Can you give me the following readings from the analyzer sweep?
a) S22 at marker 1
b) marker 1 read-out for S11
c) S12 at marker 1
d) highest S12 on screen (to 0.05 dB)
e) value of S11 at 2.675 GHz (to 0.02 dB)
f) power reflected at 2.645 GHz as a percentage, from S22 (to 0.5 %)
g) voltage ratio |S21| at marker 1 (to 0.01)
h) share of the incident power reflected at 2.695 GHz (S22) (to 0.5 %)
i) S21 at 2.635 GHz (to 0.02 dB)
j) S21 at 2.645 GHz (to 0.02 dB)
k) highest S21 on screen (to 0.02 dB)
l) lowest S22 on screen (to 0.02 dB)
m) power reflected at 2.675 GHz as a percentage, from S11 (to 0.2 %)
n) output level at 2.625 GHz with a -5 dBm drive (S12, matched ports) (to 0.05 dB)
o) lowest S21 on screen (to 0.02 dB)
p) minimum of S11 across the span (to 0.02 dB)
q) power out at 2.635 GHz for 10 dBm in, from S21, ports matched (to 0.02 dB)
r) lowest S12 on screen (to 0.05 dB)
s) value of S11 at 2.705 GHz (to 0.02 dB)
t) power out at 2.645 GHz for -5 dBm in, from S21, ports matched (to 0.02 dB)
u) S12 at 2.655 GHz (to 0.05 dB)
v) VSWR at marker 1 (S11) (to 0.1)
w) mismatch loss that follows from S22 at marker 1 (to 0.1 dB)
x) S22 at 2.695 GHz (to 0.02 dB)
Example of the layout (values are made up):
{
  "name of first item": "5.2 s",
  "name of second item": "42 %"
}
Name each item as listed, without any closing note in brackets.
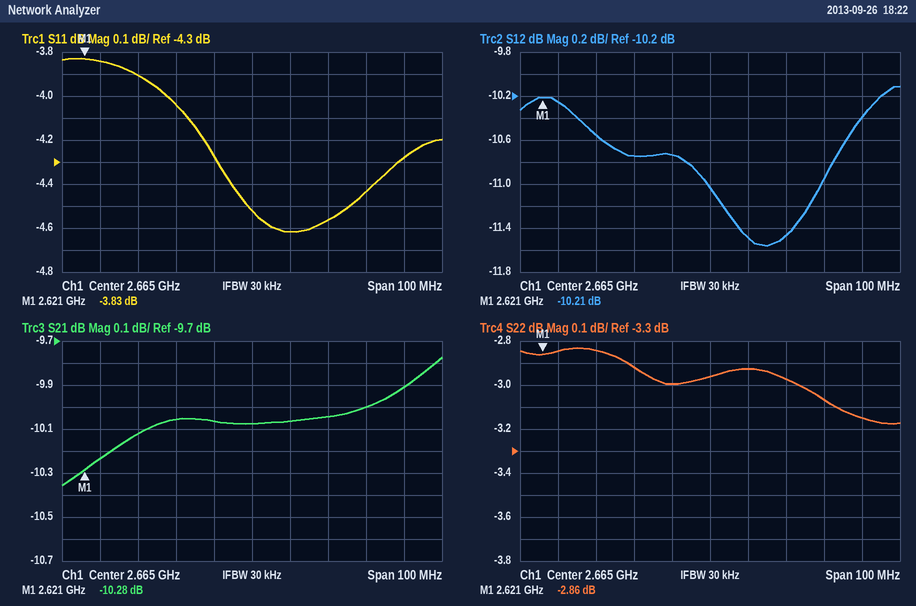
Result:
{
  "S22 at marker 1": "-2.86 dB",
  "marker 1 read-out for S11": "-3.83 dB",
  "S12 at marker 1": "-10.21 dB",
  "highest S12 on screen": "-10.10 dB",
  "value of S11 at 2.675 GHz": "-4.62 dB",
  "power reflected at 2.645 GHz as a percentage, from S22": "51.0 %",
  "voltage ratio |S21| at marker 1": "0.31",
  "share of the incident power reflected at 2.695 GHz (S22)": "49.5 %",
  "S21 at 2.635 GHz": "-10.12 dB",
  "S21 at 2.645 GHz": "-10.06 dB",
  "highest S21 on screen": "-9.78 dB",
  "lowest S22 on screen": "-3.18 dB",
  "power reflected at 2.675 GHz as a percentage, from S11": "34.6 %",
  "output level at 2.625 GHz with a -5 dBm drive (S12, matched ports)": "-15.25 dBm",
  "lowest S21 on screen": "-10.36 dB",
  "minimum of S11 across the span": "-4.62 dB",
  "power out at 2.635 GHz for 10 dBm in, from S21, ports matched": "-0.12 dBm",
  "lowest S12 on screen": "-11.55 dB",
  "value of S11 at 2.705 GHz": "-4.28 dB",
  "power out at 2.645 GHz for -5 dBm in, from S21, ports matched": "-15.06 dBm",
  "S12 at 2.655 GHz": "-10.75 dB",
  "VSWR at marker 1 (S11)": "4.6",
  "mismatch loss that follows from S22 at marker 1": "3.2 dB",
  "S22 at 2.695 GHz": "-3.06 dB"
}
